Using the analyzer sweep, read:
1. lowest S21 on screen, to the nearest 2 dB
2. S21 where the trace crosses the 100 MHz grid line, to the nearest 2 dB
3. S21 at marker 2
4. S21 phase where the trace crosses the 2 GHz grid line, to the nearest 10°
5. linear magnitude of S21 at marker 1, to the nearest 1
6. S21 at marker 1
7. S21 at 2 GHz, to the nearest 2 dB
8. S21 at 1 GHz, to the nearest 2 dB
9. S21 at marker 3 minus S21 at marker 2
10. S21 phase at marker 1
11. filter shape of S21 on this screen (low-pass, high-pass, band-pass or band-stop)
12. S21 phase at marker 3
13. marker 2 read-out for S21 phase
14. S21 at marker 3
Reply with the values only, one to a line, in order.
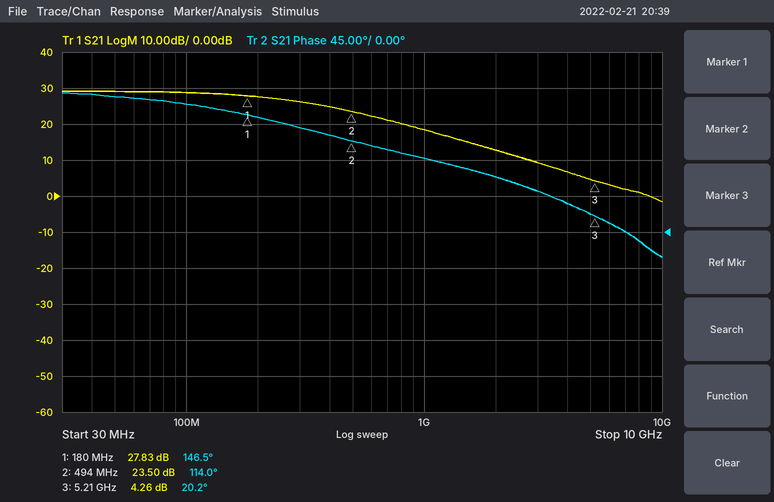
-2 dB
28 dB
23.50 dB
70°
25
27.83 dB
12 dB
18 dB
-19.24 dB
146.5°
low-pass
20.2°
114.0°
4.26 dB
